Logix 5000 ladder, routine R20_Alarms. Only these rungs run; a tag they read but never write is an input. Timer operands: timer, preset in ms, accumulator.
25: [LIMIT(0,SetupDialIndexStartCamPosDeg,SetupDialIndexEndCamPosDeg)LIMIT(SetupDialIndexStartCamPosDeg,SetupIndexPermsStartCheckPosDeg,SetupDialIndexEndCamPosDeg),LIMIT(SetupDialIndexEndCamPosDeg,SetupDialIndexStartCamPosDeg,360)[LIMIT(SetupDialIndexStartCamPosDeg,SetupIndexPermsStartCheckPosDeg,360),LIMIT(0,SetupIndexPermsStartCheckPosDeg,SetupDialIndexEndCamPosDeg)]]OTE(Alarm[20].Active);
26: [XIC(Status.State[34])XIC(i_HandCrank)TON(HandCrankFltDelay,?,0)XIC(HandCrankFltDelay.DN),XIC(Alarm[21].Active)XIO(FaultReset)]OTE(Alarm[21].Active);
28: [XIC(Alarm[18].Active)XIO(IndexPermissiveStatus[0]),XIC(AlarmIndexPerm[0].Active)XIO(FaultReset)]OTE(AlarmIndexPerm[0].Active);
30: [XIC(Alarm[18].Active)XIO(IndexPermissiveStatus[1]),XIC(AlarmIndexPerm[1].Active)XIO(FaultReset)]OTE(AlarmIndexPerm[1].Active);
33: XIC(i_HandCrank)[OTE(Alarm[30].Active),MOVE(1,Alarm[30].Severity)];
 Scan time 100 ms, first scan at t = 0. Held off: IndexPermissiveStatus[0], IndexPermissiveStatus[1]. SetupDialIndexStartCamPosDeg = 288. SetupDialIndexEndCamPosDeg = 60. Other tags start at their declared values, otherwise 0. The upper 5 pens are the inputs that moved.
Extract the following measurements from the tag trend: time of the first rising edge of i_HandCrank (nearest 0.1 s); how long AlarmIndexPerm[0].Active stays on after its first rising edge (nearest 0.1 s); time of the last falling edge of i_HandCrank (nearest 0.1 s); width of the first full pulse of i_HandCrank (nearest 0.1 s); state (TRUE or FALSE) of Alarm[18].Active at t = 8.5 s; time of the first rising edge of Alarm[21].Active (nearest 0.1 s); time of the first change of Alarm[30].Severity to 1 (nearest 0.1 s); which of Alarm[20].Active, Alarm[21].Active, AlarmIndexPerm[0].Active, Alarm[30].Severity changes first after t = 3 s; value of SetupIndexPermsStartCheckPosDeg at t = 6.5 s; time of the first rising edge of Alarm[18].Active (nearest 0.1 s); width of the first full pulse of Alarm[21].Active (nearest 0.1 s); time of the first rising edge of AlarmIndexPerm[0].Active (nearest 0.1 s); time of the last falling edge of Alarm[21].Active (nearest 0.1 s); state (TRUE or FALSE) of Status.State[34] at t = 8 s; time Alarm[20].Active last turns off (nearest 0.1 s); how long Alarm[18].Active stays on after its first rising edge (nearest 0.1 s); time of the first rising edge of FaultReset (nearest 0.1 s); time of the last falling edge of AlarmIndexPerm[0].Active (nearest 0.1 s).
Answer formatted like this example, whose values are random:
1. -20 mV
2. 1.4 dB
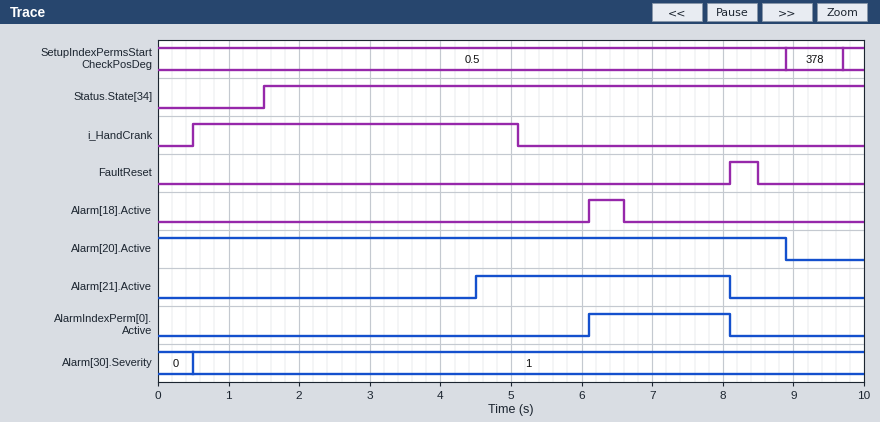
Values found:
1. 0.5 s
2. 2.0 s
3. 5.1 s
4. 4.6 s
5. FALSE
6. 4.5 s
7. 0.5 s
8. Alarm[21].Active
9. 0.5
10. 6.1 s
11. 3.6 s
12. 6.1 s
13. 8.1 s
14. TRUE
15. 8.9 s
16. 0.5 s
17. 8.1 s
18. 8.1 s
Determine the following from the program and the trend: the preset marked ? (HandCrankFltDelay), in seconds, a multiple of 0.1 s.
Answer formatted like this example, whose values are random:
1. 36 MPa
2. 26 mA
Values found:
1. 3.0 s
